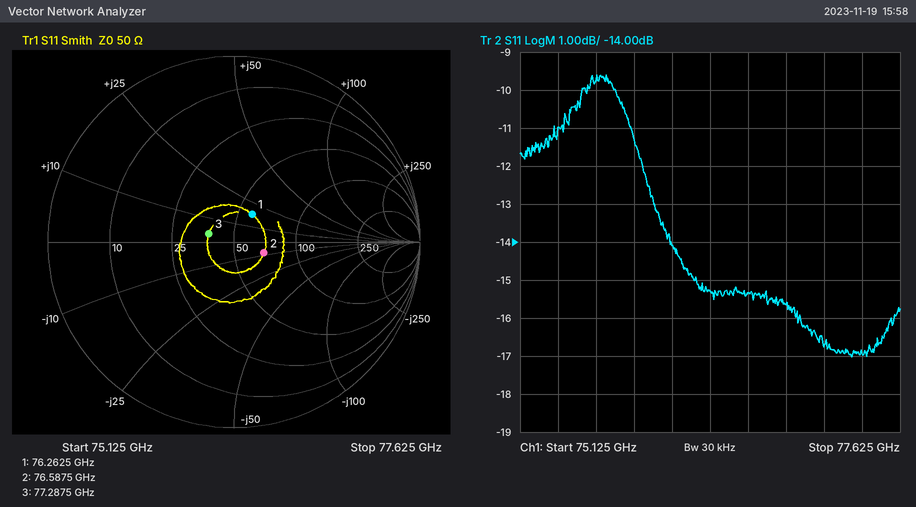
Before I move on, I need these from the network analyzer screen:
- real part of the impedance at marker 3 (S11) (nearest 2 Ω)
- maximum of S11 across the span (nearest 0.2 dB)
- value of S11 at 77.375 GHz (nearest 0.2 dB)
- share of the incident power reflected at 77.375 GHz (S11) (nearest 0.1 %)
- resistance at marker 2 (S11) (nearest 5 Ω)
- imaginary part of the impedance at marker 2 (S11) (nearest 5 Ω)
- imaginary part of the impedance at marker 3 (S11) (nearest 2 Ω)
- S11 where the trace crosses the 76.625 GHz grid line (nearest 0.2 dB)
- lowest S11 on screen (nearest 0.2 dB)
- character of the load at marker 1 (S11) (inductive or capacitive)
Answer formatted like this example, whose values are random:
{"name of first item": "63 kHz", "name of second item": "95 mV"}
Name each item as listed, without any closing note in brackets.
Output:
{"real part of the impedance at marker 3 (S11)": "38 Ω", "maximum of S11 across the span": "-9.6 dB", "value of S11 at 77.375 GHz": "-17.0 dB", "share of the incident power reflected at 77.375 GHz (S11)": "2.0 %", "resistance at marker 2 (S11)": "70 Ω", "imaginary part of the impedance at marker 2 (S11)": "-10 Ω", "imaginary part of the impedance at marker 3 (S11)": "+4 Ω", "S11 where the trace crosses the 76.625 GHz grid line": "-15.4 dB", "lowest S11 on screen": "-17.0 dB", "character of the load at marker 1 (S11)": "inductive"}
